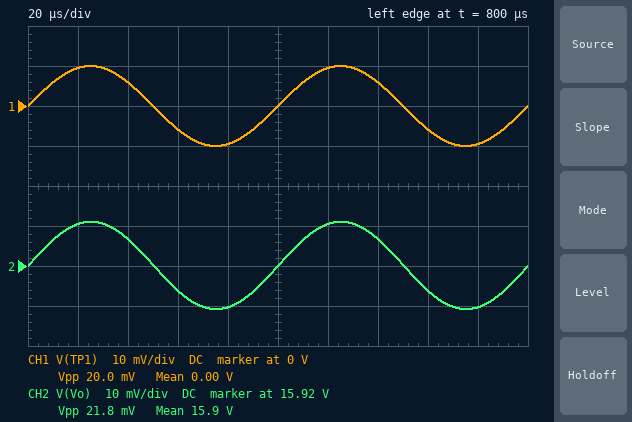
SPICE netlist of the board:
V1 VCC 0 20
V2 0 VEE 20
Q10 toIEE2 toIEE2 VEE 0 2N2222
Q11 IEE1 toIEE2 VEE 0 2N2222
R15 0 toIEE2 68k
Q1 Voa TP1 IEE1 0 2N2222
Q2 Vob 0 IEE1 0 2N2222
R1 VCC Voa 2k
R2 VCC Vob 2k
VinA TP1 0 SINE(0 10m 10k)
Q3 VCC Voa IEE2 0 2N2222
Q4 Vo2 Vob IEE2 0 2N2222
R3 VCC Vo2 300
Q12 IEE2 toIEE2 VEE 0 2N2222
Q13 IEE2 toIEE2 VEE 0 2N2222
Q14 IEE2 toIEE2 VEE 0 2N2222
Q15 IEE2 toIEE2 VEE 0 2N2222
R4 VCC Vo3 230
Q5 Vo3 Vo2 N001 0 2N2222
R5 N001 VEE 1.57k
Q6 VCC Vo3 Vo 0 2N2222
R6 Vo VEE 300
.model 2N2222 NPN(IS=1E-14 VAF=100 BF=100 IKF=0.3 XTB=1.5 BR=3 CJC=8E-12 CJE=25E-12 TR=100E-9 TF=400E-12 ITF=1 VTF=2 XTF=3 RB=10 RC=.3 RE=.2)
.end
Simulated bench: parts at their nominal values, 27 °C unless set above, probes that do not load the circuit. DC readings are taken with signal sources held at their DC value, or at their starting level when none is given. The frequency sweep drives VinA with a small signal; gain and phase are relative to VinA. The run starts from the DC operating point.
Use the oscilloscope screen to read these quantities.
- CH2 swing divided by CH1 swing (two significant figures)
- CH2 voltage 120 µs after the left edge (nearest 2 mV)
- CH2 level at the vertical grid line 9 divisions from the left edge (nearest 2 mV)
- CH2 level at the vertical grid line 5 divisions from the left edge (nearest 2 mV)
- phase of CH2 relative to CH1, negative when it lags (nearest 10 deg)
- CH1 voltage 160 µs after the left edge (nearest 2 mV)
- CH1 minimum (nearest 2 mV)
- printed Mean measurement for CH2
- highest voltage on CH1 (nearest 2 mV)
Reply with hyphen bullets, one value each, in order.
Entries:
- 1.1
- 15.930 V
- 15.910 V
- 15.920 V
- 0 deg
- -6 mV
- -10 mV
- 15.9 V
- 10 mV
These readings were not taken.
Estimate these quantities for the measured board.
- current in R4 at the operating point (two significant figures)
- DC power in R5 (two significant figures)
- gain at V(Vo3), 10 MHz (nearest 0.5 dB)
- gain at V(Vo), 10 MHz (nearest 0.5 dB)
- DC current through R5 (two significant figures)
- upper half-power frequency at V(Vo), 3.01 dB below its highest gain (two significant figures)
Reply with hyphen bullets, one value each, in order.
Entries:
- 14 mA
- 860 mW
- -10.5 dB
- -10.5 dB
- 23 mA
- 670 kHz
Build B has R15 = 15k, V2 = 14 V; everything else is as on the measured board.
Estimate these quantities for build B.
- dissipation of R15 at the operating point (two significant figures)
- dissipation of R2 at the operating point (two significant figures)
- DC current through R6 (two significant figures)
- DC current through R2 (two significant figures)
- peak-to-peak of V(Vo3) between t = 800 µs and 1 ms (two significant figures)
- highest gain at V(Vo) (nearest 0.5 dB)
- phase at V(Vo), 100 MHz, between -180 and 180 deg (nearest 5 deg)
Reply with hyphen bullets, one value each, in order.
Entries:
- 12 mW
- 1.1 mW
- 100 mA
- 740 µA
- 63 mV
- 10.0 dB
- 30 deg
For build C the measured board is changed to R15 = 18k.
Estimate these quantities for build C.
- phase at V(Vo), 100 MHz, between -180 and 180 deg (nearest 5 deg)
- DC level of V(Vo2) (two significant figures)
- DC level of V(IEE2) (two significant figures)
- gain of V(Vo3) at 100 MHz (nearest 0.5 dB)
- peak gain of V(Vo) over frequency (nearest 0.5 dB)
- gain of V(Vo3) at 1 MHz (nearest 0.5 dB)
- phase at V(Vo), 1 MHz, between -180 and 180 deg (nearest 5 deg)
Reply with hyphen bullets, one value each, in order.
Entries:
- 35 deg
- 17 V
- 18 V
- -6.5 dB
- 12.0 dB
- 7.5 dB
- -50 deg
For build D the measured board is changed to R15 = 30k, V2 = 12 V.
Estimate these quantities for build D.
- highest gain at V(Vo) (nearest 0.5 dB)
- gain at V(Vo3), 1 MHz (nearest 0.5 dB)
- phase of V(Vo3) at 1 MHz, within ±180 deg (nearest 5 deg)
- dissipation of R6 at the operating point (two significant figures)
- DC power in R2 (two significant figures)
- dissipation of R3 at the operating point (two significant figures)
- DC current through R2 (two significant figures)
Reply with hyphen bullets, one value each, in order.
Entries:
- 2.5 dB
- -2.0 dB
- -50 deg
- 2.7 W
- 760 µW
- 12 mW
- 620 µA
